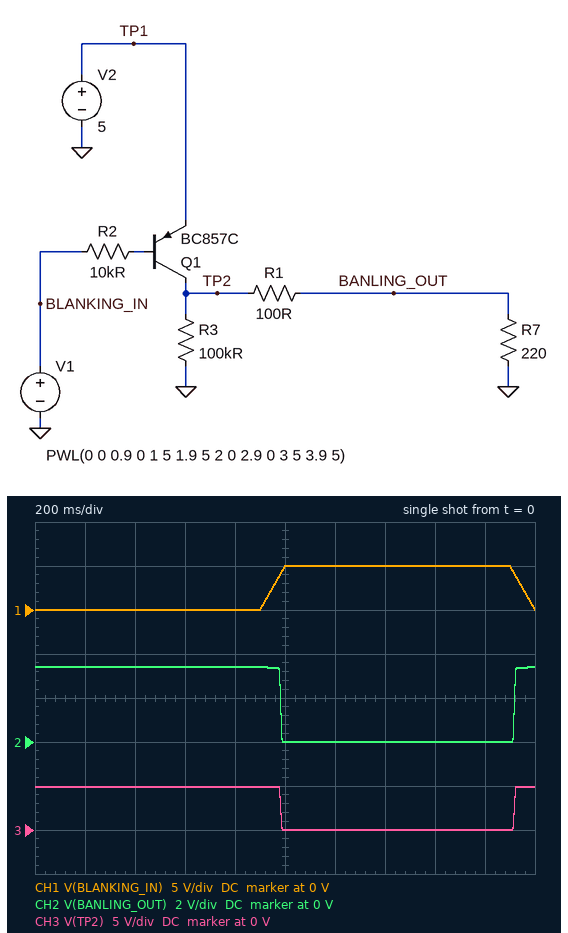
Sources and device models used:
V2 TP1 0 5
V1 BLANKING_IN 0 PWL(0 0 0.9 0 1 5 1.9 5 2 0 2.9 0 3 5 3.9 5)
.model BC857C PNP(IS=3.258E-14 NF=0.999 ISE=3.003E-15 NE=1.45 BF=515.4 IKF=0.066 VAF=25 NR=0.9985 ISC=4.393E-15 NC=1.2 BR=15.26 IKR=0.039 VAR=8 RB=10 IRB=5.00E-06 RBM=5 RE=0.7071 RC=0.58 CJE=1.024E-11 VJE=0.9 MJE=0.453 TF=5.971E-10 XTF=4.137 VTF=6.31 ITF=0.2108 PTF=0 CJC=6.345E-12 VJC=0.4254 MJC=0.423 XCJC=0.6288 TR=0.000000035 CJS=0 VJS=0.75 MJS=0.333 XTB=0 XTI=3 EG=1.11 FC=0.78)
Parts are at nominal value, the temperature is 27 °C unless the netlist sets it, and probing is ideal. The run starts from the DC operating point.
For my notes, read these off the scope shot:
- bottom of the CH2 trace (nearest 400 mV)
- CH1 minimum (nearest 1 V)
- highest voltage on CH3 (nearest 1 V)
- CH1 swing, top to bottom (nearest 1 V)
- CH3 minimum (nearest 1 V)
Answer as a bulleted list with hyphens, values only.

- 0 V
- 0 V
- 5 V
- 5 V
- 0 V
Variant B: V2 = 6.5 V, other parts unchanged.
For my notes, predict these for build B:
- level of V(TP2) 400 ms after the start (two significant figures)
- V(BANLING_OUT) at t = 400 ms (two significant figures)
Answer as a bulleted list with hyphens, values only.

- 6.4 V
- 4.4 V
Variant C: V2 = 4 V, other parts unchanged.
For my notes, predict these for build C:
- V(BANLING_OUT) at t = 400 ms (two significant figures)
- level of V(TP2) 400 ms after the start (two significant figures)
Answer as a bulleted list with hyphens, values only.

- 2.7 V
- 3.9 V
